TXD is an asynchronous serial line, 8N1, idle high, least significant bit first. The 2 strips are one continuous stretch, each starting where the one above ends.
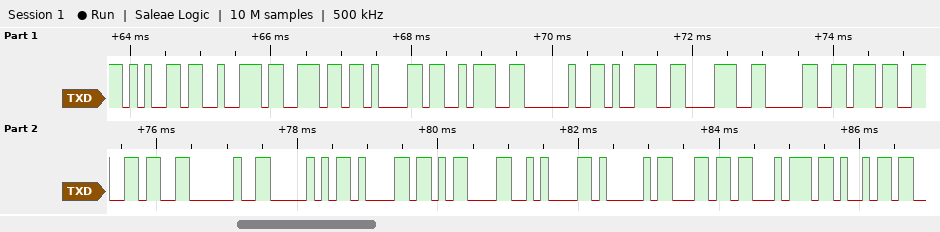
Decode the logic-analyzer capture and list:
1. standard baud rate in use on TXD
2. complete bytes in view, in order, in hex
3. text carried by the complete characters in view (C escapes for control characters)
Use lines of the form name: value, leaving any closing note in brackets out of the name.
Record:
standard baud rate in use on TXD: 9600 baud
complete bytes in view, in order, in hex: 65 72 6E 61 3A 20 39 38 30 37 36 20 50 61 0D 0A 41 6C 74 69
text carried by the complete characters in view: "erna: 98076 Pa\r\nAlti"
